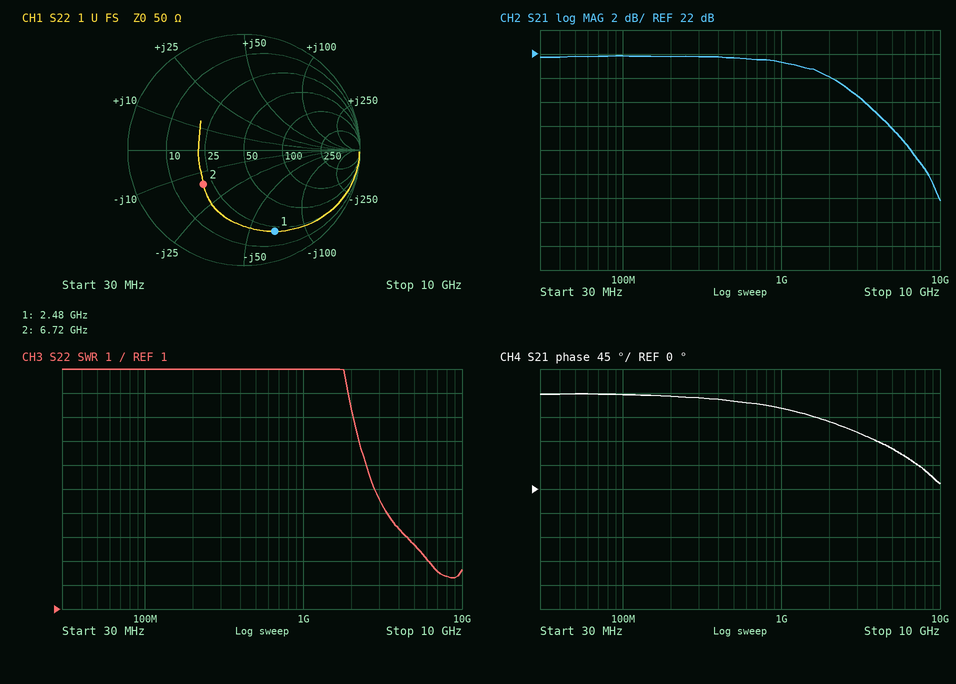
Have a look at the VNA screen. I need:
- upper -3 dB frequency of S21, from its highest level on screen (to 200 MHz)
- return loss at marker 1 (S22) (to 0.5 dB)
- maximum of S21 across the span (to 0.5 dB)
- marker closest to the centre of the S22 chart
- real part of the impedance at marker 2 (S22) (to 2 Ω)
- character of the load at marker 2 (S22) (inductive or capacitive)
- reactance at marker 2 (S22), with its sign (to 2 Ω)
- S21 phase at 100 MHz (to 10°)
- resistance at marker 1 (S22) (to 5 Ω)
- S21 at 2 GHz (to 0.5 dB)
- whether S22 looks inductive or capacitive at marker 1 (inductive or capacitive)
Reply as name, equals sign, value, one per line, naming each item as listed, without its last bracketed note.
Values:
upper -3 dB frequency of S21, from its highest level on screen = 2.8 GHz
return loss at marker 1 (S22) = 2.5 dB
maximum of S21 across the span = 22.0 dB
marker closest to the centre of the S22 chart = marker 2
real part of the impedance at marker 2 (S22) = 20 Ω
character of the load at marker 2 (S22) = capacitive
reactance at marker 2 (S22), with its sign = -16 Ω
S21 phase at 100 MHz = 180°
resistance at marker 1 (S22) = 20 Ω
S21 at 2 GHz = 20.0 dB
whether S22 looks inductive or capacitive at marker 1 = capacitive
